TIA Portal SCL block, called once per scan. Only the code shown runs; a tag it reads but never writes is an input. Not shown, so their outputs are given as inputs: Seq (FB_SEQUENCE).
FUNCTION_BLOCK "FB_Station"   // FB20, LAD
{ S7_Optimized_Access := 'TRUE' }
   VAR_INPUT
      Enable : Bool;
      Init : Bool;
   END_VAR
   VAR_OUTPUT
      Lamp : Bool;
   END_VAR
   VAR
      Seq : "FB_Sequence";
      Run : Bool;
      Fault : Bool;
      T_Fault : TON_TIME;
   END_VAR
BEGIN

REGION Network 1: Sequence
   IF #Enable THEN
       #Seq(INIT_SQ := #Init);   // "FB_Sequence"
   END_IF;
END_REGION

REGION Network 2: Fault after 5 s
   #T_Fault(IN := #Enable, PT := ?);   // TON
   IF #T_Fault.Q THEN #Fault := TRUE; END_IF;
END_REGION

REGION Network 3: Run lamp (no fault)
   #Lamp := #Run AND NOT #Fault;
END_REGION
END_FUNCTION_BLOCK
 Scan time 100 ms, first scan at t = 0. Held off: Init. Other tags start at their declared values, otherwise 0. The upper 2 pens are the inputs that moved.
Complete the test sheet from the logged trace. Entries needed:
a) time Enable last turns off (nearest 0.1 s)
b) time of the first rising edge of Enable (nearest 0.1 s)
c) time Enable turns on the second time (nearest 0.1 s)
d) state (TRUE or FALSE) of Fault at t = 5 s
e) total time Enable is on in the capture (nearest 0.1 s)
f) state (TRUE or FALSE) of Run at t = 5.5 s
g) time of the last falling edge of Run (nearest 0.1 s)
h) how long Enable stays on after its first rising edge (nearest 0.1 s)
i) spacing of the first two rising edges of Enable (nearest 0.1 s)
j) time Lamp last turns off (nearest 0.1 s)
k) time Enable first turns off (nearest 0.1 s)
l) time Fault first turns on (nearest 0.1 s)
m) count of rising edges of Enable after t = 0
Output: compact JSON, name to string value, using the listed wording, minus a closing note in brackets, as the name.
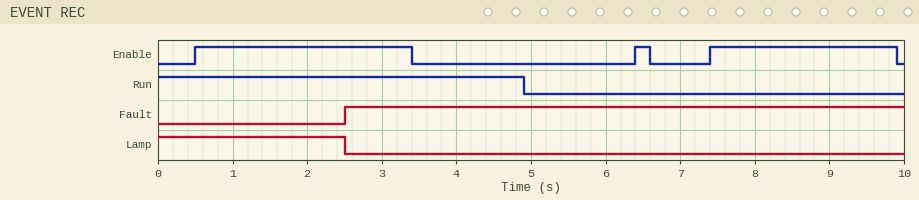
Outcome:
{"time Enable last turns off": "9.9 s", "time of the first rising edge of Enable": "0.5 s", "time Enable turns on the second time": "6.4 s", "state (TRUE or FALSE) of Fault at t = 5 s": "TRUE", "total time Enable is on in the capture": "5.6 s", "state (TRUE or FALSE) of Run at t = 5.5 s": "FALSE", "time of the last falling edge of Run": "4.9 s", "how long Enable stays on after its first rising edge": "2.9 s", "spacing of the first two rising edges of Enable": "5.9 s", "time Lamp last turns off": "2.5 s", "time Enable first turns off": "3.4 s", "time Fault first turns on": "2.5 s", "count of rising edges of Enable after t = 0": "3"}
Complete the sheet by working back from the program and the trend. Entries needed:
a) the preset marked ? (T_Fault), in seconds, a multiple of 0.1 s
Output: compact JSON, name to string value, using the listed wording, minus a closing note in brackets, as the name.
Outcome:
{"the preset marked ? (T_Fault), in seconds, a multiple of 0.1 s": "2.0 s"}
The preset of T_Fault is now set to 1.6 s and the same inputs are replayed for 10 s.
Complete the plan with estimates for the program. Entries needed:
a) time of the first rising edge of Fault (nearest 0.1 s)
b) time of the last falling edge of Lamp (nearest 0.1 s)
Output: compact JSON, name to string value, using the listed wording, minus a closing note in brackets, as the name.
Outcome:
{"time of the first rising edge of Fault": "2.1 s", "time of the last falling edge of Lamp": "2.1 s"}
